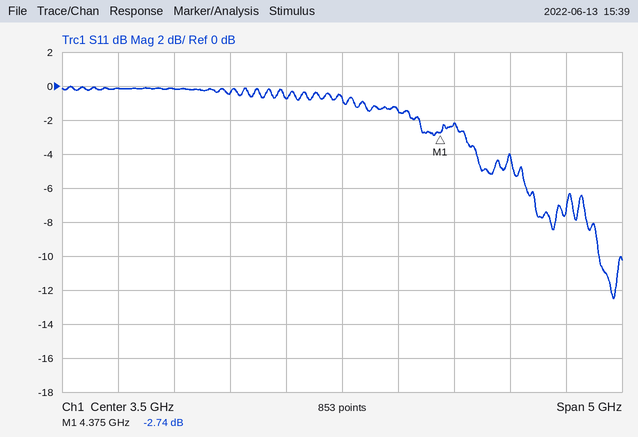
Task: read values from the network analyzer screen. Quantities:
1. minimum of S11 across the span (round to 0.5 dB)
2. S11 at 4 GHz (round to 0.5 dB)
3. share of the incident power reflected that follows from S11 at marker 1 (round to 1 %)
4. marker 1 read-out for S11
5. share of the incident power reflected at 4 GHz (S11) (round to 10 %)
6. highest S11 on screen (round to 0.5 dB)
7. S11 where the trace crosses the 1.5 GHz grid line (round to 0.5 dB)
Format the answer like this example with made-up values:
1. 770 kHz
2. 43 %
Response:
1. -12.5 dB
2. -1.5 dB
3. 53 %
4. -2.74 dB
5. 70 %
6. 0.0 dB
7. 0.0 dB
